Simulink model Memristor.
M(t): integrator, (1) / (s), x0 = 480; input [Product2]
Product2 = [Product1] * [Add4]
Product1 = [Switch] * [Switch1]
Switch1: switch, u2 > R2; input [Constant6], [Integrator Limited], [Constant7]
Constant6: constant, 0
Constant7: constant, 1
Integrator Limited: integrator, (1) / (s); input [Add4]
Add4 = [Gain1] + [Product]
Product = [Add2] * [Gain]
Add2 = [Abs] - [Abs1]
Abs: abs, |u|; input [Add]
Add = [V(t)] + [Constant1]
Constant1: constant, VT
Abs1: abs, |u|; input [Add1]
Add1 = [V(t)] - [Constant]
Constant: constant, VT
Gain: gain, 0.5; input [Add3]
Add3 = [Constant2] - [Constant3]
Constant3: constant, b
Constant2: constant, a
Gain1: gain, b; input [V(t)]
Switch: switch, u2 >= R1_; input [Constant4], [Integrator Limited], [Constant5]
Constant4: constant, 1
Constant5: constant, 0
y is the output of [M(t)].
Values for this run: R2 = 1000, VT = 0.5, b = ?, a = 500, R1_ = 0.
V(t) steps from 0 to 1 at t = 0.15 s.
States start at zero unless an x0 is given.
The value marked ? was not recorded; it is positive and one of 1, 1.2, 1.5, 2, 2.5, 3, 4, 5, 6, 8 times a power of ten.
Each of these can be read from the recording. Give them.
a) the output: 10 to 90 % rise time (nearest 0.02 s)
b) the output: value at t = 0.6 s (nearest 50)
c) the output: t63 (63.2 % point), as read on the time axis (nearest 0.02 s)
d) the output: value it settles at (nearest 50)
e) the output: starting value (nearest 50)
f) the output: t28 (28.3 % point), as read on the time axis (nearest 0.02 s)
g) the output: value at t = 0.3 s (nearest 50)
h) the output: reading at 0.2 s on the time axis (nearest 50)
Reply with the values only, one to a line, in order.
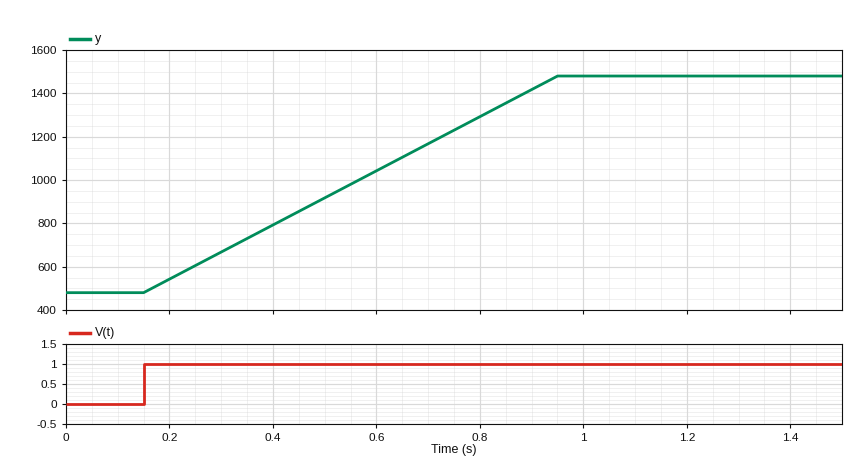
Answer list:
0.64 s
1050
0.66 s
1500
500
0.38 s
650
550
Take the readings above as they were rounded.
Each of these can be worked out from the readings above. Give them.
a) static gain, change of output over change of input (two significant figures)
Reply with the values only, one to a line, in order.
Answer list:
1000
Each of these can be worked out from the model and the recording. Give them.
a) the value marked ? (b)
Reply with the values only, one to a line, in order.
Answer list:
2000
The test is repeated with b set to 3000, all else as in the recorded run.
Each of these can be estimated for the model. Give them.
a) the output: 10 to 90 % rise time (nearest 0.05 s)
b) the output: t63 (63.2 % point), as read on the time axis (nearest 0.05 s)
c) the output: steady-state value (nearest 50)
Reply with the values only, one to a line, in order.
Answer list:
0.45 s
0.50 s
1500
